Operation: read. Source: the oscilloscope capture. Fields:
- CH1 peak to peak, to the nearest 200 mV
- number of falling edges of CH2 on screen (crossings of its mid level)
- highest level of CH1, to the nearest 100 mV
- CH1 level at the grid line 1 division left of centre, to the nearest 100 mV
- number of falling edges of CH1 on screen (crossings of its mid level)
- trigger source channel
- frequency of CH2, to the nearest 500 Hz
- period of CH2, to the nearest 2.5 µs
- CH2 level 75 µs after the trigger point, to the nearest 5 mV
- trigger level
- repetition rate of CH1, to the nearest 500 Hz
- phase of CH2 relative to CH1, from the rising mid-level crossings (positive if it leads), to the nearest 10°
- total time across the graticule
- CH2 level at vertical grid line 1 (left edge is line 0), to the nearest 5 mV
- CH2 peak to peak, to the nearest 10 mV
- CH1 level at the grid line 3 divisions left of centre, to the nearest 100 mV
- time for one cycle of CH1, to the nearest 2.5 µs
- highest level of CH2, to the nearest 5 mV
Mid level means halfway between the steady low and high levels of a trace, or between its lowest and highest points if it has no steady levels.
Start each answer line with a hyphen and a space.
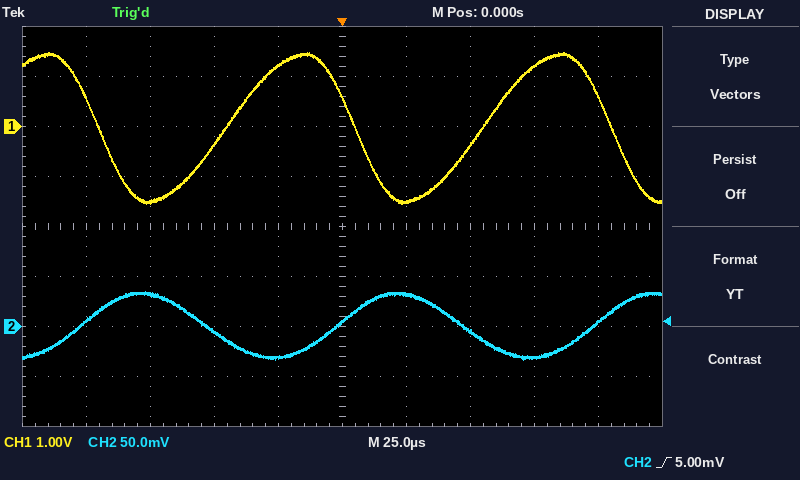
- 3.0 V
- 2
- 1.5 V
- 1.2 V
- 3
- CH2
- 10.0 kHz
- 100.0 µs
- -30 mV
- 5.00 mV
- 10.0 kHz
- -160°
- 250 µs
- 5 mV
- 70 mV
- -1.5 V
- 100.0 µs
- 35 mV
